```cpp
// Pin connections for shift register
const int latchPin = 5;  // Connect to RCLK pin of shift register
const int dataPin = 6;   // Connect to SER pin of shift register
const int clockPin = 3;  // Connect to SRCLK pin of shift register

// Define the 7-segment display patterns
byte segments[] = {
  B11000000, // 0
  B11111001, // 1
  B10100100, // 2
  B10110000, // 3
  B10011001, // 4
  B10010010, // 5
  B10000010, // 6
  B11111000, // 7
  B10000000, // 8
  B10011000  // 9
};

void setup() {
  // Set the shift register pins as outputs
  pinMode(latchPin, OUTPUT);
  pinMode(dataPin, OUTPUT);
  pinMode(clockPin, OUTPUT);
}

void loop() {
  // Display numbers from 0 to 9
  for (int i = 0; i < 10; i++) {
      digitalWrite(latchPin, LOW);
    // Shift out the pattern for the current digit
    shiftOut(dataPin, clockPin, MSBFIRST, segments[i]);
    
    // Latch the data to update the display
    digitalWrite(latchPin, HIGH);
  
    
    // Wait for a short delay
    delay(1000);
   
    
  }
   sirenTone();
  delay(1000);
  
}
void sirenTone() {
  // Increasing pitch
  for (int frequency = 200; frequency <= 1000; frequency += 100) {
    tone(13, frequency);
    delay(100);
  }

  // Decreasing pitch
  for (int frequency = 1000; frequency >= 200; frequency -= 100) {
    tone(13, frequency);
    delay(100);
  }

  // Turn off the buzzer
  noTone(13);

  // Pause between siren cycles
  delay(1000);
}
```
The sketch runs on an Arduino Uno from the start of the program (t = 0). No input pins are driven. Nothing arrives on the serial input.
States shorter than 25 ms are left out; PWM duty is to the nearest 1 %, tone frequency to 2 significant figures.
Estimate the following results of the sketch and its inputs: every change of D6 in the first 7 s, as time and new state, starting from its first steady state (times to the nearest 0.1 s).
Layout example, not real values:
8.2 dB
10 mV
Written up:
0 s low; 1 s high; 2 s low; 4 s high; 5 s low
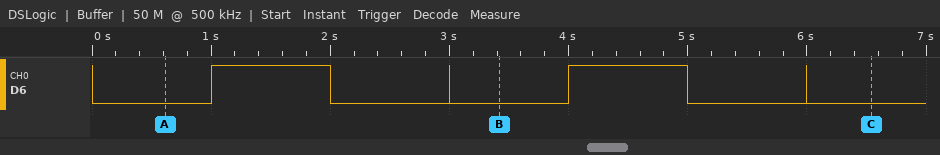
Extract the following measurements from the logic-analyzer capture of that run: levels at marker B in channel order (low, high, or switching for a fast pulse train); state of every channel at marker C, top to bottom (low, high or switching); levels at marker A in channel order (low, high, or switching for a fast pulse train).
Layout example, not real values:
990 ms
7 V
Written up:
D6 low
D6 low
D6 low
